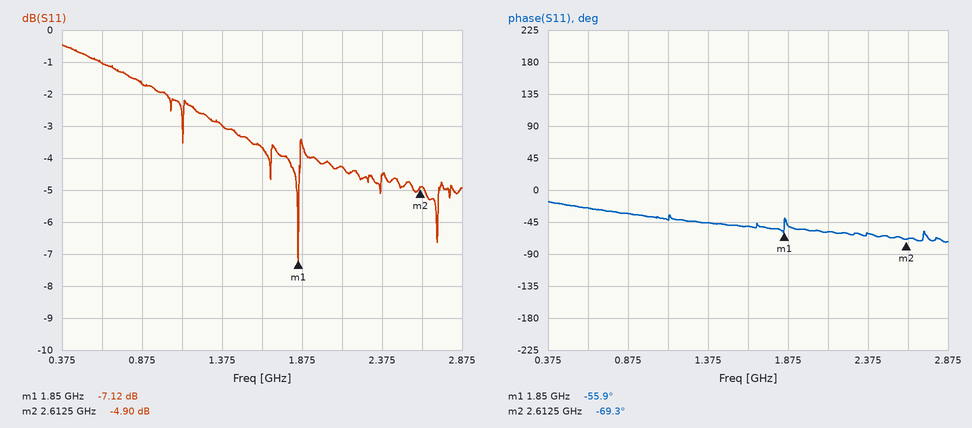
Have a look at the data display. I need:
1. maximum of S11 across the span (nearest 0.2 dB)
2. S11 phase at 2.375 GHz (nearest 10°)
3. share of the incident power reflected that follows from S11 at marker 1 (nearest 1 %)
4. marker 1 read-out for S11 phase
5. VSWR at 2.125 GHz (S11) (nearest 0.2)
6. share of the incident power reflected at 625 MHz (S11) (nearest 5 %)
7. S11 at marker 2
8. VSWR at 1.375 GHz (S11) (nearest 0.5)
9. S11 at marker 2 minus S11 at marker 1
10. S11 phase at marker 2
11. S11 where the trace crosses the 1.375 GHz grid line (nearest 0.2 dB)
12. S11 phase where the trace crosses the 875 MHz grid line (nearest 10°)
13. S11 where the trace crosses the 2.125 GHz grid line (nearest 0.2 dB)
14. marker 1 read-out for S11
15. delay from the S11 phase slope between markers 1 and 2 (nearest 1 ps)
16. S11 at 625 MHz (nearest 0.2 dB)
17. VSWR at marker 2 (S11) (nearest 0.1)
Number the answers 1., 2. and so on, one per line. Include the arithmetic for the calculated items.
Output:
1. -0.4 dB
2. -60°
3. 10^(-7.12/10) ≈ 19 %
4. -55.9°
5. |Γ| = 10^(-4.2/20) = 0.6166; VSWR = (1 + 0.6166)/(1 − 0.6166) ≈ 4.2
6. 10^(-1/10) ≈ 79.4 %, so 80 % to the nearest 5 %
7. -4.90 dB
8. |Γ| = 10^(-3/20) = 0.7079; VSWR = (1 + 0.7079)/(1 − 0.7079) ≈ 5.85, so 6.0 to the nearest 0.5
9. -4.9 − (-7.12) = 2.22 dB
10. -69.3°
11. -3.0 dB
12. -30°
13. -4.2 dB
14. -7.12 dB
15. −(-69.3° − (-55.9°))/(360° × 762.5 MHz) ≈ 49 ps
16. -1.0 dB
17. (1 + 0.5689)/(1 − 0.5689) ≈ 3.6
